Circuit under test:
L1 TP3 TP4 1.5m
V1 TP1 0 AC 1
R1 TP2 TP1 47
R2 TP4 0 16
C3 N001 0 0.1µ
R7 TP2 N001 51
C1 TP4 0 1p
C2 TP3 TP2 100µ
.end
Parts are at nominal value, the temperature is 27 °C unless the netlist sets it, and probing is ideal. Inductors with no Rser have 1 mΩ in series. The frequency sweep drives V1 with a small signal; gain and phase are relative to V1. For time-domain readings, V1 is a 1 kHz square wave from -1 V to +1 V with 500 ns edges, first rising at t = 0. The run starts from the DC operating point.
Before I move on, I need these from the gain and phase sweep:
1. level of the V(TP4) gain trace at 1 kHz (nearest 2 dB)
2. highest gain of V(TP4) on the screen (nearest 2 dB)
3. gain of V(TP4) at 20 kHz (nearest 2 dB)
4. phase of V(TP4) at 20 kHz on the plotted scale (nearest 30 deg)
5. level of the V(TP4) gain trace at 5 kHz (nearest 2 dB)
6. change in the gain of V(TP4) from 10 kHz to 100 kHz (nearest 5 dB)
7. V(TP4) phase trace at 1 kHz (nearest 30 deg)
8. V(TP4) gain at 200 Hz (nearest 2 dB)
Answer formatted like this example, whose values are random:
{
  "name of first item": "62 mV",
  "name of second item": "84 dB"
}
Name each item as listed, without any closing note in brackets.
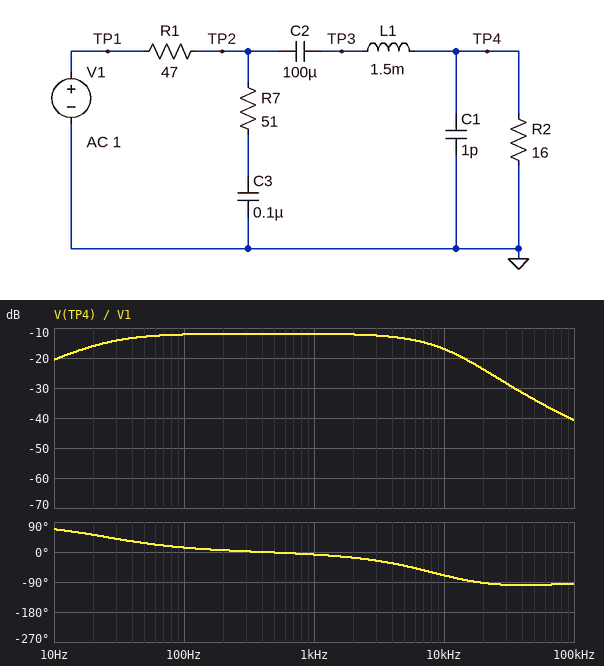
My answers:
{
  "level of the V(TP4) gain trace at 1 kHz": "-12 dB",
  "highest gain of V(TP4) on the screen": "-12 dB",
  "gain of V(TP4) at 20 kHz": "-24 dB",
  "phase of V(TP4) at 20 kHz on the plotted scale": "-90 deg",
  "level of the V(TP4) gain trace at 5 kHz": "-14 dB",
  "change in the gain of V(TP4) from 10 kHz to 100 kHz": "-25 dB",
  "V(TP4) phase trace at 1 kHz": "0 deg",
  "V(TP4) gain at 200 Hz": "-12 dB"
}
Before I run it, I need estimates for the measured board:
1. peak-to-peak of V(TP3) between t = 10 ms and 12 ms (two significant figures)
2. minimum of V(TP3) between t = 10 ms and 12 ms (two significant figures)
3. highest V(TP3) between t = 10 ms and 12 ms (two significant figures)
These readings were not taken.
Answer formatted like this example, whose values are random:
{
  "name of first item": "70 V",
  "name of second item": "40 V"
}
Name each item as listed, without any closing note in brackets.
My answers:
{
  "peak-to-peak of V(TP3) between t = 10 ms and 12 ms": "2.3 V",
  "minimum of V(TP3) between t = 10 ms and 12 ms": "-1.1 V",
  "highest V(TP3) between t = 10 ms and 12 ms": "1.2 V"
}
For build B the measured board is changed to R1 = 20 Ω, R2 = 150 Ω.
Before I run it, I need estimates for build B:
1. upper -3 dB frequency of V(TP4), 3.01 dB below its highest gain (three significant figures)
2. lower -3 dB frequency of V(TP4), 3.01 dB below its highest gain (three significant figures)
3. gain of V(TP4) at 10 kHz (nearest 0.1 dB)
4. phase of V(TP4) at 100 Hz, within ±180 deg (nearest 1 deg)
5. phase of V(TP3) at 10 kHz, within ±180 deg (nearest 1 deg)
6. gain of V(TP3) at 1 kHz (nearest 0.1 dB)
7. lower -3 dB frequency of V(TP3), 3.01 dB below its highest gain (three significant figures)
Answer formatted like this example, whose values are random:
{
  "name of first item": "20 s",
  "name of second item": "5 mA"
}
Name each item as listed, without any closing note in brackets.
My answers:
{
  "upper -3 dB frequency of V(TP4), 3.01 dB below its highest gain": "15.5 kHz",
  "lower -3 dB frequency of V(TP4), 3.01 dB below its highest gain": "9.36 Hz",
  "gain of V(TP4) at 10 kHz": "-2.5 dB",
  "phase of V(TP4) at 100 Hz, within ±180 deg": "5 deg",
  "phase of V(TP3) at 10 kHz, within ±180 deg": "-3 deg",
  "gain of V(TP3) at 1 kHz": "-1.1 dB",
  "lower -3 dB frequency of V(TP3), 3.01 dB below its highest gain": "9.40 Hz"
}
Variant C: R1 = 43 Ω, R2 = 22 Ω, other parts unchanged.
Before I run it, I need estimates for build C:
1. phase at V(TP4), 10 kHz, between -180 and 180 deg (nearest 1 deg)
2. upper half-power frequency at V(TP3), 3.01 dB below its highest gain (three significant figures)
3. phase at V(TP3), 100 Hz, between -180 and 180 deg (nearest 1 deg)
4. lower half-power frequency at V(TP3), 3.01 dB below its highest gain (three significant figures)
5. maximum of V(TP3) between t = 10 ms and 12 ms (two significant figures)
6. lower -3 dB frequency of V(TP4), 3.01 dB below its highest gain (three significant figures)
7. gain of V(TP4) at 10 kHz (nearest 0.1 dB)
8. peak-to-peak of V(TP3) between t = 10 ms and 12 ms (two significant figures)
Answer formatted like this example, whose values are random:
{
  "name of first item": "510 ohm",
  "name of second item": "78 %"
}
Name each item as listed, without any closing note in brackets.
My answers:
{
  "phase at V(TP4), 10 kHz, between -180 and 180 deg": "-68 deg",
  "upper half-power frequency at V(TP3), 3.01 dB below its highest gain": "56.2 kHz",
  "phase at V(TP3), 100 Hz, between -180 and 180 deg": "15 deg",
  "lower half-power frequency at V(TP3), 3.01 dB below its highest gain": "4.04 kHz",
  "maximum of V(TP3) between t = 10 ms and 12 ms": "1.2 V",
  "lower -3 dB frequency of V(TP4), 3.01 dB below its highest gain": "24.4 Hz",
  "gain of V(TP4) at 10 kHz": "-14.4 dB",
  "peak-to-peak of V(TP3) between t = 10 ms and 12 ms": "2.2 V"
}
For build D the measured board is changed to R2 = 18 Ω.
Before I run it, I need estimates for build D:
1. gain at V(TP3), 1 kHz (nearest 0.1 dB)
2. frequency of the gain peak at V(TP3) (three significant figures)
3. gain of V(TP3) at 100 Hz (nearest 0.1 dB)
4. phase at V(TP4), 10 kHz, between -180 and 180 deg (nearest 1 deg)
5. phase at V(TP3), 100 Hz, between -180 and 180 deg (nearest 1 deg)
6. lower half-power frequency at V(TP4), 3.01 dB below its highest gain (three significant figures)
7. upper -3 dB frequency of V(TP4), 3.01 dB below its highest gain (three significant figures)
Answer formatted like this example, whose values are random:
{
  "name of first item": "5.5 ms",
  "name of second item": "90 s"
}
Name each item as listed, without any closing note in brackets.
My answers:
{
  "gain at V(TP3), 1 kHz": "-10.1 dB",
  "frequency of the gain peak at V(TP3)": "11.6 kHz",
  "gain of V(TP3) at 100 Hz": "-11.4 dB",
  "phase at V(TP4), 10 kHz, between -180 and 180 deg": "-69 deg",
  "phase at V(TP3), 100 Hz, between -180 and 180 deg": "16 deg",
  "lower half-power frequency at V(TP4), 3.01 dB below its highest gain": "24.4 Hz",
  "upper -3 dB frequency of V(TP4), 3.01 dB below its highest gain": "7.34 kHz"
}
